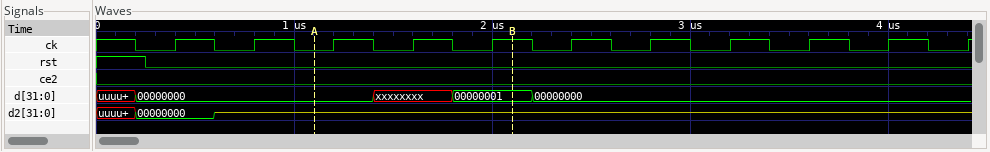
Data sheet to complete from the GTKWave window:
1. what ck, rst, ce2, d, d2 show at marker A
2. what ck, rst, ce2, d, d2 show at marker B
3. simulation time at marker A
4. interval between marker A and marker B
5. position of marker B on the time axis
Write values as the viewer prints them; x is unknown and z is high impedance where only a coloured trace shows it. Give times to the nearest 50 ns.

ck=0, rst=0, ce2=0, d=00000000, d2=z
ck=1, rst=0, ce2=0, d=00000001, d2=z
1100 ns
1000 ns
2100 ns
